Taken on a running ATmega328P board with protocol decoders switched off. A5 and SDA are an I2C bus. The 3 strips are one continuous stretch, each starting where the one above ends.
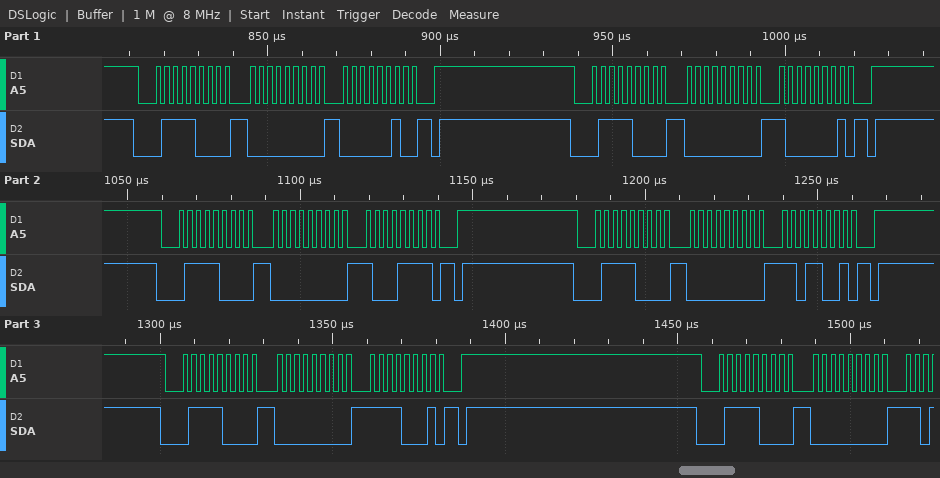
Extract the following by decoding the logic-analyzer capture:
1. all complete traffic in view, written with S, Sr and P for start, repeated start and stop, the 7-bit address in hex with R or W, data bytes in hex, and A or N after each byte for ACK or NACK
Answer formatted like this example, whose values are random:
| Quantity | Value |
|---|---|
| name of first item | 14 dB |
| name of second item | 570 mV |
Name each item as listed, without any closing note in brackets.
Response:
| Quantity | Value |
|---|---|
| all complete traffic in view, written with S, Sr and P for start, repeated start and stop, the 7-bit address in hex with R or W, data bytes in hex, and A or N after each byte for ACK or NACK | S 3CW A 00 A 02 A P S 3CW A 00 A 81 A P S 3CW A 00 A 8F A P S 3CW A 00 A D9 A P S 3CW A 00 A F1 A P S 3CW A 00 A |
